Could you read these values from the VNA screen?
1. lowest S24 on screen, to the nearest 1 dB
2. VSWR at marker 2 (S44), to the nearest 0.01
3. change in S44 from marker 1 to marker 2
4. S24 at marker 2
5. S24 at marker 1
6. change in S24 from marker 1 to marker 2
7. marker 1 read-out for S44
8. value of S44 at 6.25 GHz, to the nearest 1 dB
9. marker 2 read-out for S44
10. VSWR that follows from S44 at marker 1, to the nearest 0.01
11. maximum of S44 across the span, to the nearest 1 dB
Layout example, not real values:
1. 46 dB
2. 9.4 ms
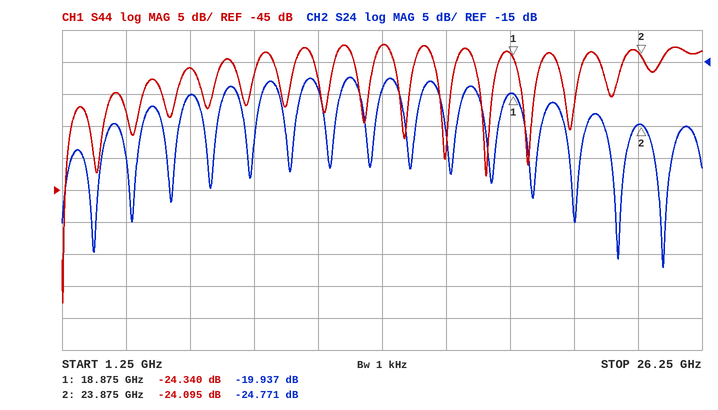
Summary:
1. -47 dB
2. 1.13
3. 0.245 dB
4. -24.771 dB
5. -19.937 dB
6. -4.834 dB
7. -24.340 dB
8. -26 dB
9. -24.095 dB
10. 1.13
11. -22 dB
